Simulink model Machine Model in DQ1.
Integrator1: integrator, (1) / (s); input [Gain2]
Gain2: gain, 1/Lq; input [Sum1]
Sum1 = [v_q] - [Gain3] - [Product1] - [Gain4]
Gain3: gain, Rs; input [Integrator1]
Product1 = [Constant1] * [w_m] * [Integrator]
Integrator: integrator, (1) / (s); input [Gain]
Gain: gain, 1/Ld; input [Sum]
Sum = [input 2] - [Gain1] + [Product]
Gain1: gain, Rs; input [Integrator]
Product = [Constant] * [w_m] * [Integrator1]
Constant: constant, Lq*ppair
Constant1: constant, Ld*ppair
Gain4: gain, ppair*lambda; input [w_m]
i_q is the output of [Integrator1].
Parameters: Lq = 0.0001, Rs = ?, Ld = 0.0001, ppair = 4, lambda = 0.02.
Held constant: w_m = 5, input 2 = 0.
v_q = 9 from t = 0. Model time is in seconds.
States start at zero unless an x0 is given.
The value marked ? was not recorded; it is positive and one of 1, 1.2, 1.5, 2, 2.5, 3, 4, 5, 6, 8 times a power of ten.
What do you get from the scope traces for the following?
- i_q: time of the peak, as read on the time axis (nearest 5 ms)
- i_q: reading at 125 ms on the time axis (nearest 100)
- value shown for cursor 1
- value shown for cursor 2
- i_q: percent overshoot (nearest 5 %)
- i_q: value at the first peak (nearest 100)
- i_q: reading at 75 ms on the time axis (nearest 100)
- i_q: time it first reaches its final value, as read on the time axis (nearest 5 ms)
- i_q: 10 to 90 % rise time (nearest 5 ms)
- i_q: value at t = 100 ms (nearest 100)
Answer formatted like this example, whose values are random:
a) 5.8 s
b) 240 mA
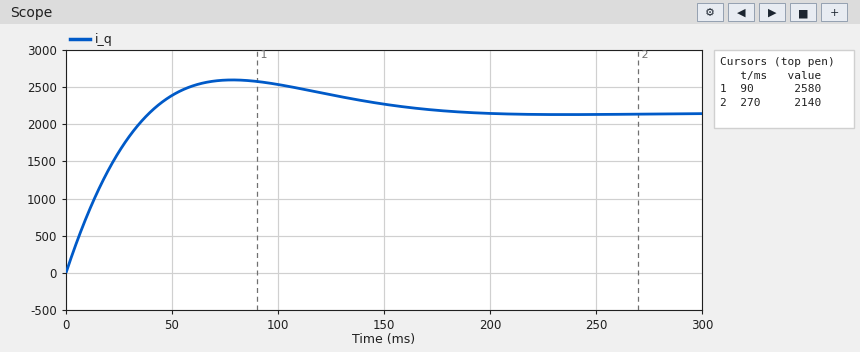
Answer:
a) 80 ms
b) 2400
c) 2580
d) 2140
e) 20 %
f) 2600
g) 2600
h) 40 ms
i) 30 ms
j) 2500
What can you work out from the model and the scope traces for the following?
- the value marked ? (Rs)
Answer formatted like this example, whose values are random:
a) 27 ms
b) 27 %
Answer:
a) 0.002
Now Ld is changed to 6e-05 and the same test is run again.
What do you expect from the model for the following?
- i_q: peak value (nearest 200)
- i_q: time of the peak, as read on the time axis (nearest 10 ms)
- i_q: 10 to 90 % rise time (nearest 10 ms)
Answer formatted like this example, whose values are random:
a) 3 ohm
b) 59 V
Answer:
a) 2800
b) 100 ms
c) 50 ms
